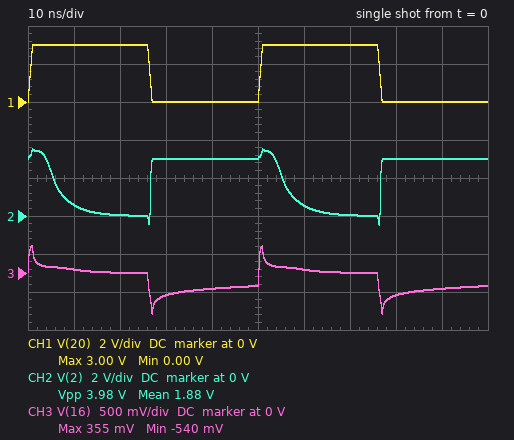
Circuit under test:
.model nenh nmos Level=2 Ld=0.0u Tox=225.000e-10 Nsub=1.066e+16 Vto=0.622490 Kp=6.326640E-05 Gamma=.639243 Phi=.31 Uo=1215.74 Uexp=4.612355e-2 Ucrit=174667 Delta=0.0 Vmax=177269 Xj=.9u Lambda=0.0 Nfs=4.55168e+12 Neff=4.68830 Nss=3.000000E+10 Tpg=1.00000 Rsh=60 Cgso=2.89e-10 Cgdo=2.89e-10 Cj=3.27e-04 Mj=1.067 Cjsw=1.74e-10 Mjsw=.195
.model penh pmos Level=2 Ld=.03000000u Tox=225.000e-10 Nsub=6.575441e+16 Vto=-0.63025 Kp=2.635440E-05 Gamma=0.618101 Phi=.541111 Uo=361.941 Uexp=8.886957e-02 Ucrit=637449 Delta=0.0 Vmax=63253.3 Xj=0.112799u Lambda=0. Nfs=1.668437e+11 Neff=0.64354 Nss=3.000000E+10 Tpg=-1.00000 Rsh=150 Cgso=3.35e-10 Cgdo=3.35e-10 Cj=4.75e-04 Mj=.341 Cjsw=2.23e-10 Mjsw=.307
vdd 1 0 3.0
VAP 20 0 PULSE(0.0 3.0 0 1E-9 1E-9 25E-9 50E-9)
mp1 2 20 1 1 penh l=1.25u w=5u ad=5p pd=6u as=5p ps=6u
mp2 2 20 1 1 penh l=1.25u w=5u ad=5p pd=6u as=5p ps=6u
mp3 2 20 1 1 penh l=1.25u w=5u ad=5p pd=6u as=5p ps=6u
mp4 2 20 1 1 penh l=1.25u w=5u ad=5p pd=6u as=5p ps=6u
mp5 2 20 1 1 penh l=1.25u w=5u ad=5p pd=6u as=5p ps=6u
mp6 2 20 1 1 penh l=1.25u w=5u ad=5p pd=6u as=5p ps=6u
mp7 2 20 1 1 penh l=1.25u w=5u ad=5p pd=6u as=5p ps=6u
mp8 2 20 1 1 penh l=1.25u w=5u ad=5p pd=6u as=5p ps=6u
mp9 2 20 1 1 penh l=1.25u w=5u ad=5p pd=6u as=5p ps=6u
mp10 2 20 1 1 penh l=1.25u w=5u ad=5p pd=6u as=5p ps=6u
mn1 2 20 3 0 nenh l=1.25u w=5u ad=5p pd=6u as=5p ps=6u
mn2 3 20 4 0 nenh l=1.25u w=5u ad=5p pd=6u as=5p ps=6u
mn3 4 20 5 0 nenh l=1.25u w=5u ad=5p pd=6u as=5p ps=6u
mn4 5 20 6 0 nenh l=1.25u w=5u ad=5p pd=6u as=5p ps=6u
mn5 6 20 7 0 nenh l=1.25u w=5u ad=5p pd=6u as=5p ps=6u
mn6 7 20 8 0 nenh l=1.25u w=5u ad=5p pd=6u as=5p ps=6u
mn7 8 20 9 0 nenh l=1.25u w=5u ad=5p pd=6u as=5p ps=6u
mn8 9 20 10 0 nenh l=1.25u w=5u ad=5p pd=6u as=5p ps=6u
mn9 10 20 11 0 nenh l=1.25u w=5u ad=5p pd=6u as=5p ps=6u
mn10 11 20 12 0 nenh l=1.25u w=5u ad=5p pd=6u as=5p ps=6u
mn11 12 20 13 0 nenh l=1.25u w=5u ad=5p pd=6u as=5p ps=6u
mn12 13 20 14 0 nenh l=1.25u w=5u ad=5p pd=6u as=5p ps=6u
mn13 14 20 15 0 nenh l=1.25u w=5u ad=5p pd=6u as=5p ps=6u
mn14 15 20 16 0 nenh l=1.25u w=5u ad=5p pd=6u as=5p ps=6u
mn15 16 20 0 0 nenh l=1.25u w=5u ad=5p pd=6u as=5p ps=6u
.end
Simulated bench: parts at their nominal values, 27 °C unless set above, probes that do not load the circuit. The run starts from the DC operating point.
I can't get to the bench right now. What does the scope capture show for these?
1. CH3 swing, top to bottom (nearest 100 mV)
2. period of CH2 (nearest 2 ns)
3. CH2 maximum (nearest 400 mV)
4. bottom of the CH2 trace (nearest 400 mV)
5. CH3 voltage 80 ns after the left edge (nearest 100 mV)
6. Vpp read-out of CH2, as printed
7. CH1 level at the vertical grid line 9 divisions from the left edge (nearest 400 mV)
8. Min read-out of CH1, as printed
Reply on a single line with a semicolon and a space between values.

900 mV; 50 ns; 3.6 V; -400 mV; -300 mV; 3.98 V; 0 V; 0.00 V
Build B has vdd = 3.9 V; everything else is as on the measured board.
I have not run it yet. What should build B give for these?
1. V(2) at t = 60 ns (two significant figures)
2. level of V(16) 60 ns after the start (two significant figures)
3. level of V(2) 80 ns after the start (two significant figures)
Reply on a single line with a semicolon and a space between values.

3.6 V; 72 mV; 3.9 V
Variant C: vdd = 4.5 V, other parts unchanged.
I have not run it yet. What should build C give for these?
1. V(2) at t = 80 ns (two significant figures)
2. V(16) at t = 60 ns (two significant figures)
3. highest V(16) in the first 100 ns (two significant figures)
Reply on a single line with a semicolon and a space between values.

4.5 V; 73 mV; 360 mV
